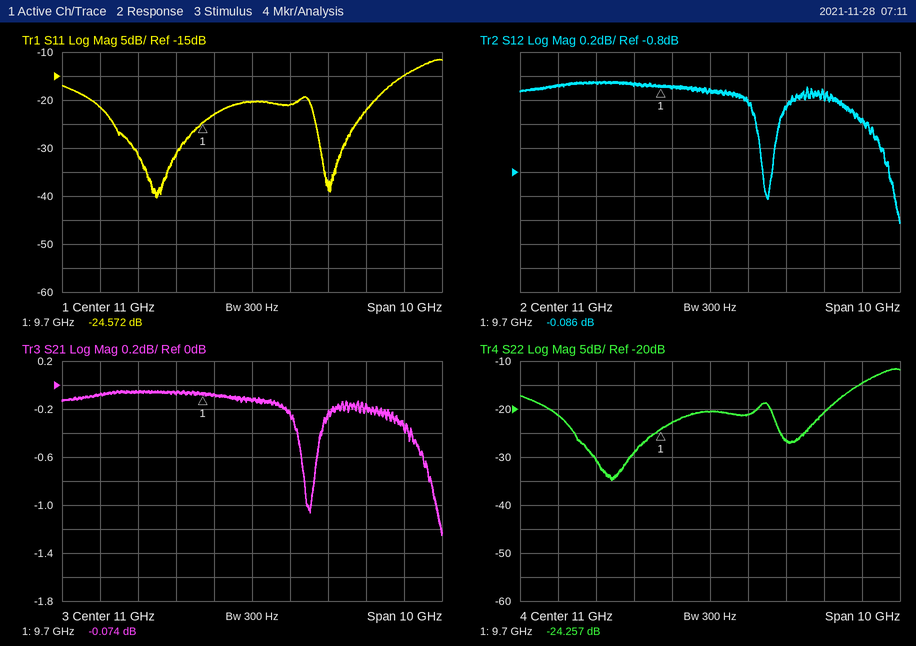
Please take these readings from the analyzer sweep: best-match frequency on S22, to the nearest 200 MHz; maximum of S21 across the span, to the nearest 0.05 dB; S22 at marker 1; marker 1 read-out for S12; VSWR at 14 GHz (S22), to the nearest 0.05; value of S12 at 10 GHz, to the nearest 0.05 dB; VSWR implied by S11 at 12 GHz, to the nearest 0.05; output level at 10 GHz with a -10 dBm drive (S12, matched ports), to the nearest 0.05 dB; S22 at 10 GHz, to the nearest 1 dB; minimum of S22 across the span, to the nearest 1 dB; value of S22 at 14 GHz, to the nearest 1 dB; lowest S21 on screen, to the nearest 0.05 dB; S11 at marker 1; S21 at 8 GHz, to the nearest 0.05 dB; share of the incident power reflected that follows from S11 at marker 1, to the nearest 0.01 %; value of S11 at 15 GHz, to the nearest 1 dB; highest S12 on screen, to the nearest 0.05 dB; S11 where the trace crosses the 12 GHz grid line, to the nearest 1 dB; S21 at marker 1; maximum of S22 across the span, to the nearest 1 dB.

8.4 GHz
-0.05 dB
-24.257 dB
-0.086 dB
1.20
-0.10 dB
1.20
-10.10 dBm
-23 dB
-35 dB
-21 dB
-1.25 dB
-24.572 dB
-0.05 dB
0.35 %
-15 dB
-0.05 dB
-21 dB
-0.074 dB
-12 dB
